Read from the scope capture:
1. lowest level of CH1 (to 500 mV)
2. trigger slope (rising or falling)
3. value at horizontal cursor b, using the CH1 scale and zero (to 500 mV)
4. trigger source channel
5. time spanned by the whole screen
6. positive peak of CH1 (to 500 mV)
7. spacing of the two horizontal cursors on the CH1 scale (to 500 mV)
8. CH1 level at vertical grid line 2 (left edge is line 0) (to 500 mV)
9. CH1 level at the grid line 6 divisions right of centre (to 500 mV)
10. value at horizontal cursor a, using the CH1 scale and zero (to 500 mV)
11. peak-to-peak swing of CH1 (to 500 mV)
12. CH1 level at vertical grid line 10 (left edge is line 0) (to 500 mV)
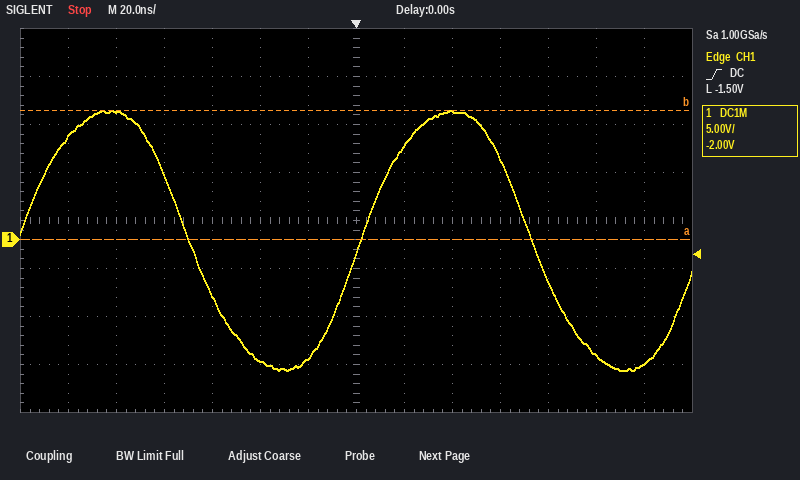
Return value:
-13.5 V
rising
13.5 V
CH1
280 ns
13.5 V
13.5 V
13.5 V
-13.0 V
0.0 V
27.0 V
8.5 V
